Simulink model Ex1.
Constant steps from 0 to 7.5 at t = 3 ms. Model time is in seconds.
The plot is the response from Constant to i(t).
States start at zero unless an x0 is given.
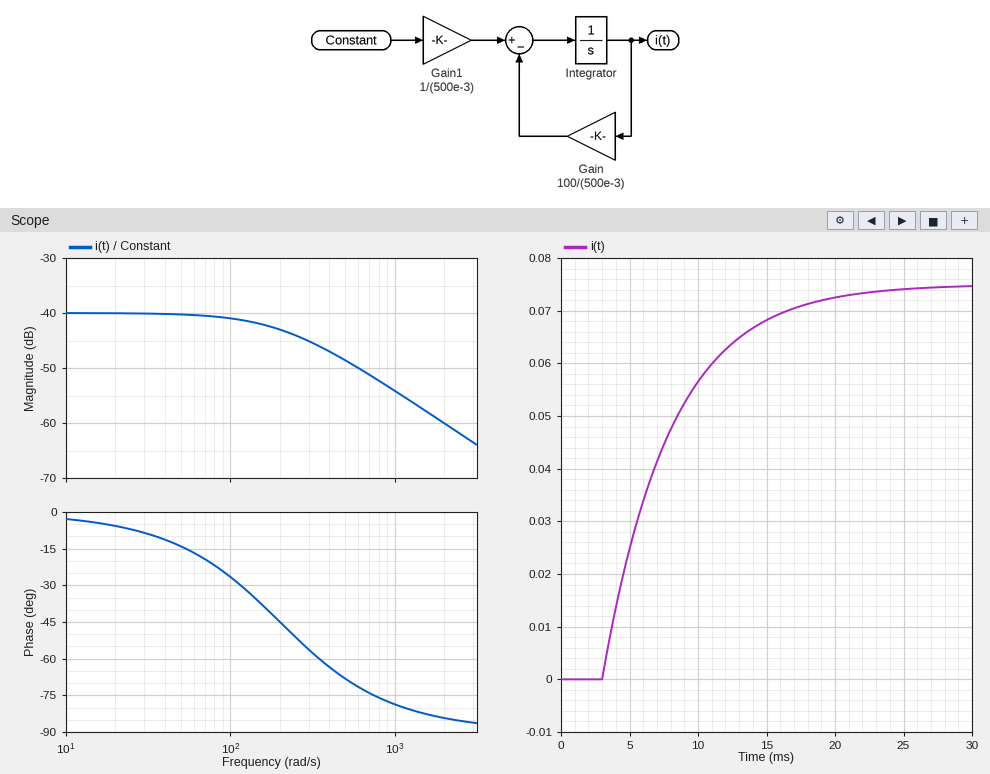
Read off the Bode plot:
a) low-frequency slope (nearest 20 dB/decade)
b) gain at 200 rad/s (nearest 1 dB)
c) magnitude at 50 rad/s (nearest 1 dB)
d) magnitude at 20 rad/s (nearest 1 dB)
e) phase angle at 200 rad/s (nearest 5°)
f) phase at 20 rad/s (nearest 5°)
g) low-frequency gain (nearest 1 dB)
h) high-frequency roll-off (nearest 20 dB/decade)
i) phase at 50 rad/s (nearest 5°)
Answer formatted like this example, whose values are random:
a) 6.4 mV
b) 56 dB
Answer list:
a) 0 dB/decade
b) -43 dB
c) -40 dB
d) -40 dB
e) -45°
f) -5°
g) -40 dB
h) -20 dB/decade
i) -15°
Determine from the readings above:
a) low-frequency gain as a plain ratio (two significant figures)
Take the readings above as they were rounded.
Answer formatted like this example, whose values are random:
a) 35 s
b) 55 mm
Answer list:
a) 0.010
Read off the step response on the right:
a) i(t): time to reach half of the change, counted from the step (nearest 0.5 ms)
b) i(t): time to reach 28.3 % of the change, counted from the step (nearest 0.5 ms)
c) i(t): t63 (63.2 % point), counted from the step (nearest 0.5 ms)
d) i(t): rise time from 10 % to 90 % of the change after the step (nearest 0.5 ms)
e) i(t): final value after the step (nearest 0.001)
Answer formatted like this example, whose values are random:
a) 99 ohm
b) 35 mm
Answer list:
a) 3.5 ms
b) 1.5 ms
c) 5.0 ms
d) 11.0 ms
e) 0.075
